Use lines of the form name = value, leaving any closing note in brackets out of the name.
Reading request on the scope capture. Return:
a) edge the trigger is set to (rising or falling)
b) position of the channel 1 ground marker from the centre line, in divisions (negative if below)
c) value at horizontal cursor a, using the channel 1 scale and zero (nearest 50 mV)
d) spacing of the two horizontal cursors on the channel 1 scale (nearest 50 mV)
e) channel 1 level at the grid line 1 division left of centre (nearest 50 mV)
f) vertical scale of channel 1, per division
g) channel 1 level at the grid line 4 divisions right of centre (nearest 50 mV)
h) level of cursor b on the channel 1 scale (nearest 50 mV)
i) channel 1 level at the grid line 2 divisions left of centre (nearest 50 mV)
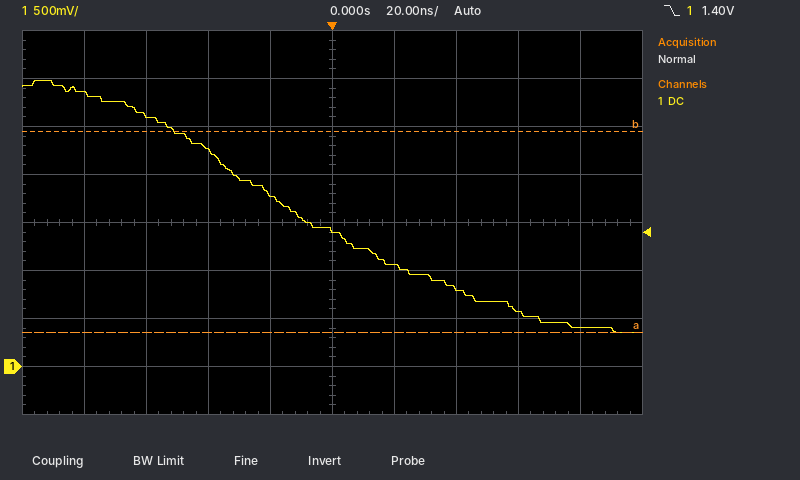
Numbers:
edge the trigger is set to = falling
position of the channel 1 ground marker from the centre line, in divisions = -3.0 div
value at horizontal cursor a, using the channel 1 scale and zero = 350 mV
spacing of the two horizontal cursors on the channel 1 scale = 2.10 V
channel 1 level at the grid line 1 division left of centre = 1.80 V
vertical scale of channel 1, per division = 500 mV
channel 1 level at the grid line 4 divisions right of centre = 400 mV
level of cursor b on the channel 1 scale = 2.45 V
channel 1 level at the grid line 2 divisions left of centre = 2.25 V
